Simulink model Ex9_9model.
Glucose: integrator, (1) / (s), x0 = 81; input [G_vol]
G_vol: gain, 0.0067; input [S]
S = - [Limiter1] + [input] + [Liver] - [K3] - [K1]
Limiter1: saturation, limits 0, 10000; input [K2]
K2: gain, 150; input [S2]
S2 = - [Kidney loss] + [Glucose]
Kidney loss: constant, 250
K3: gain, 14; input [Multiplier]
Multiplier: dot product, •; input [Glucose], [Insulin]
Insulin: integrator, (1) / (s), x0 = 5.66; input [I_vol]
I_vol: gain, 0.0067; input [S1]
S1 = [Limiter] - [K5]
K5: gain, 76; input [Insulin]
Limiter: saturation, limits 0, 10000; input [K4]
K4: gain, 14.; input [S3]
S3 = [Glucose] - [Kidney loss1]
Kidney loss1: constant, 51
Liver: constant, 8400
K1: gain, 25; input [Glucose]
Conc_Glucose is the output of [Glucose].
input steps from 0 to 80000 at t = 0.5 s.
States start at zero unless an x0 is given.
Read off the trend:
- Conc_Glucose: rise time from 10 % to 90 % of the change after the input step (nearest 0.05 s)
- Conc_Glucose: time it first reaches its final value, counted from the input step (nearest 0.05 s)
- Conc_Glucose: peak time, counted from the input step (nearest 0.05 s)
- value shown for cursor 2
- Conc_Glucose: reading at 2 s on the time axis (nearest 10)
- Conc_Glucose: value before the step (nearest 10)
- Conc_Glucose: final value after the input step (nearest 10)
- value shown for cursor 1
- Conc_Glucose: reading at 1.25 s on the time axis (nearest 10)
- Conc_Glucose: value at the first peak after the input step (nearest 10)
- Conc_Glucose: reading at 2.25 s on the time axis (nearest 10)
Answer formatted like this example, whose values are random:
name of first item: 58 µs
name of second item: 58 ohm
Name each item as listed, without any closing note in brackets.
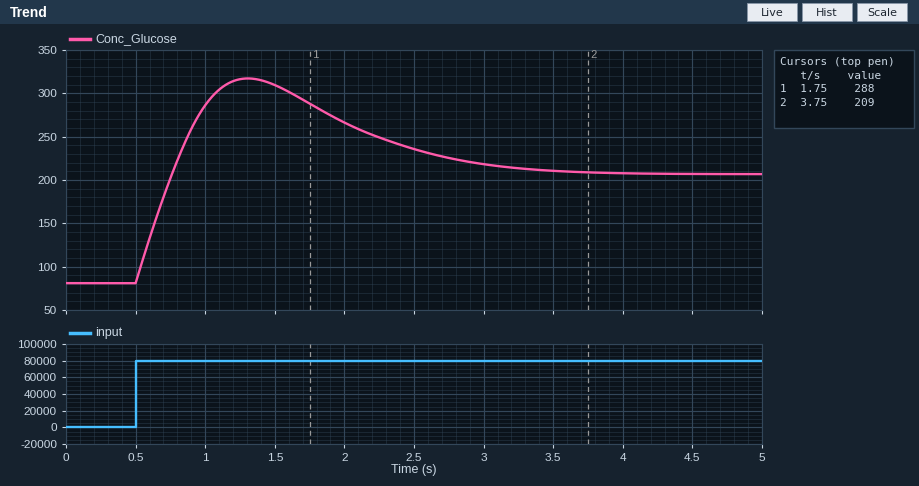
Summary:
Conc_Glucose: rise time from 10 % to 90 % of the change after the input step: 0.20 s
Conc_Glucose: time it first reaches its final value, counted from the input step: 0.25 s
Conc_Glucose: peak time, counted from the input step: 0.80 s
value shown for cursor 2: 209
Conc_Glucose: reading at 2 s on the time axis: 270
Conc_Glucose: value before the step: 80
Conc_Glucose: final value after the input step: 210
value shown for cursor 1: 288
Conc_Glucose: reading at 1.25 s on the time axis: 320
Conc_Glucose: value at the first peak after the input step: 320
Conc_Glucose: reading at 2.25 s on the time axis: 250
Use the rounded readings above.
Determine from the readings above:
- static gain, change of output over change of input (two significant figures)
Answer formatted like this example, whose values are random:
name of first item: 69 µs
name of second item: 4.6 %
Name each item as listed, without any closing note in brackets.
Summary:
static gain, change of output over change of input: 0.0016
